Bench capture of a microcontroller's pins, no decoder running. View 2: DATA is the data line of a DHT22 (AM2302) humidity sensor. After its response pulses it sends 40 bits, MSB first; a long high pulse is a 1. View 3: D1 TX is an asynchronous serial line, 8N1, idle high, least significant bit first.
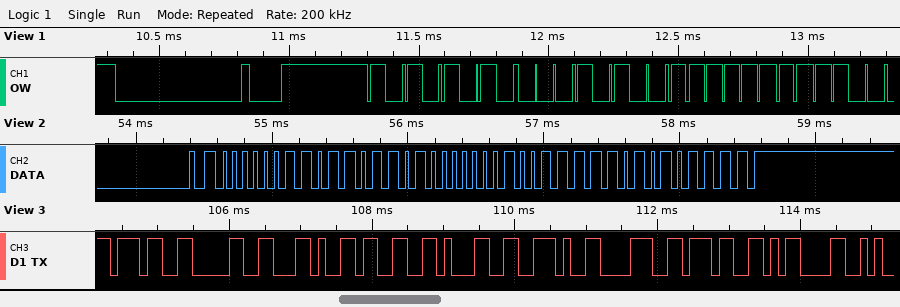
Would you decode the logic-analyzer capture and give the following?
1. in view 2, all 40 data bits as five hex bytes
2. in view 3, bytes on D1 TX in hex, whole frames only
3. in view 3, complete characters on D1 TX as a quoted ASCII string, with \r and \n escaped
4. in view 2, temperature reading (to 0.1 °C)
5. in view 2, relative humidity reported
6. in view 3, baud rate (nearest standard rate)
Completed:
03 6D 01 3E AF
37 30 2C 33 31 2E 38 37 0D
"70,31.87\r"
31.8 °C
87.7 %
9600 baud
